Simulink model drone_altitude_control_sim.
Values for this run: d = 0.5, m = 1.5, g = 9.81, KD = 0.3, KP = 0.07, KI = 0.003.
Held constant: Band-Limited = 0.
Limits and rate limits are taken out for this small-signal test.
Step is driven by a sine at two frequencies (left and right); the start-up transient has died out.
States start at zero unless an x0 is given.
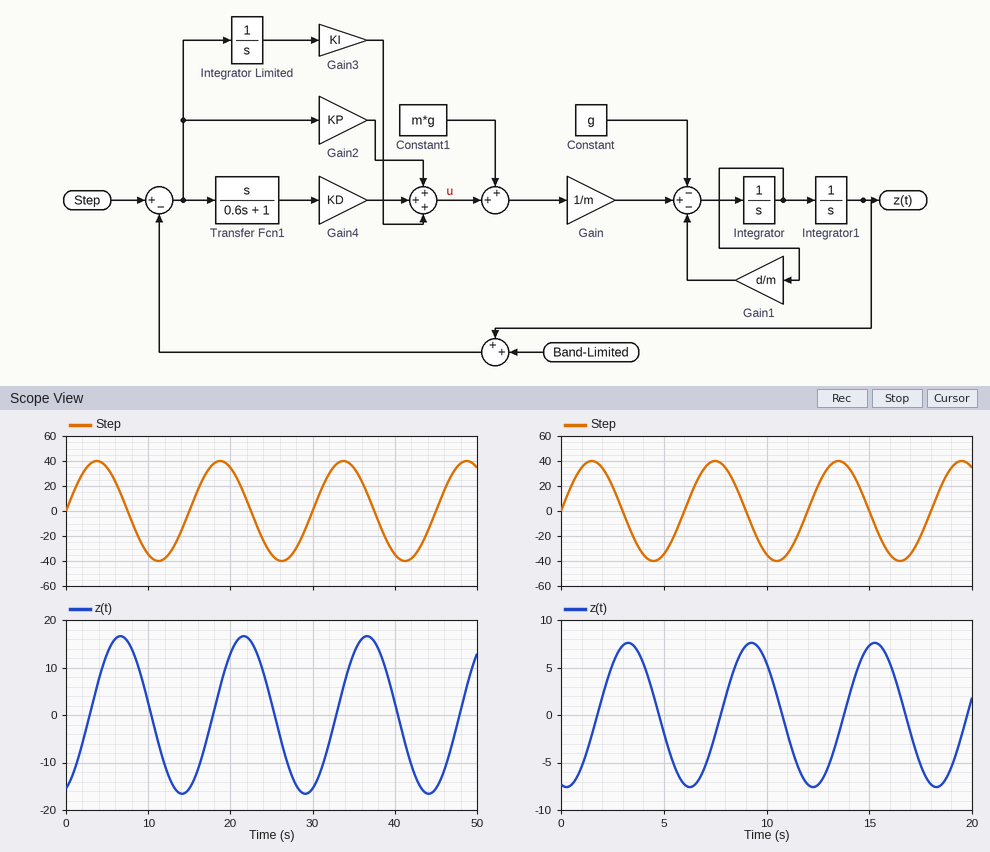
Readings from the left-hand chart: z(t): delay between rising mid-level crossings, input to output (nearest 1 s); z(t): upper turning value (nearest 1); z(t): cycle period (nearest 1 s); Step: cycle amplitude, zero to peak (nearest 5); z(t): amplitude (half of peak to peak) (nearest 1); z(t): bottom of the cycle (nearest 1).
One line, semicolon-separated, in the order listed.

3 s; 17; 15 s; 40; 17; -17
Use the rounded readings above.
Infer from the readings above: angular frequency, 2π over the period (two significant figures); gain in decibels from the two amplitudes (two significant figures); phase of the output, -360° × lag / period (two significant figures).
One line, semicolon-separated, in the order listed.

0.42 rad/s; -7.4 dB; -72°
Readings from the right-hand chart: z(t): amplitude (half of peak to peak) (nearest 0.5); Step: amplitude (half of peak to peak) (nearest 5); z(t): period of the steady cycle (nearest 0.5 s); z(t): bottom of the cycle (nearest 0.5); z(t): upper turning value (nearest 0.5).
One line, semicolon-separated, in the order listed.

7.5; 40; 6.0 s; -7.5; 7.5
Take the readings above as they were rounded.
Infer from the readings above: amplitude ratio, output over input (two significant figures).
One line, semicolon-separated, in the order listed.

0.19
